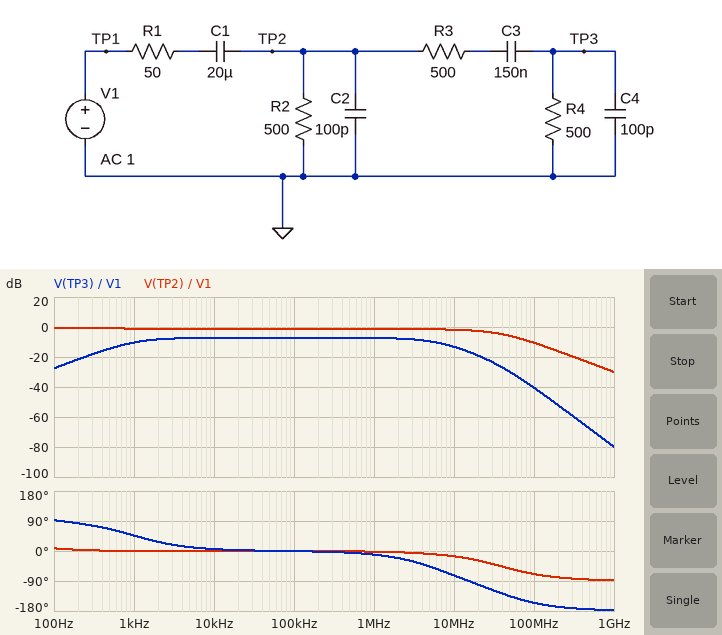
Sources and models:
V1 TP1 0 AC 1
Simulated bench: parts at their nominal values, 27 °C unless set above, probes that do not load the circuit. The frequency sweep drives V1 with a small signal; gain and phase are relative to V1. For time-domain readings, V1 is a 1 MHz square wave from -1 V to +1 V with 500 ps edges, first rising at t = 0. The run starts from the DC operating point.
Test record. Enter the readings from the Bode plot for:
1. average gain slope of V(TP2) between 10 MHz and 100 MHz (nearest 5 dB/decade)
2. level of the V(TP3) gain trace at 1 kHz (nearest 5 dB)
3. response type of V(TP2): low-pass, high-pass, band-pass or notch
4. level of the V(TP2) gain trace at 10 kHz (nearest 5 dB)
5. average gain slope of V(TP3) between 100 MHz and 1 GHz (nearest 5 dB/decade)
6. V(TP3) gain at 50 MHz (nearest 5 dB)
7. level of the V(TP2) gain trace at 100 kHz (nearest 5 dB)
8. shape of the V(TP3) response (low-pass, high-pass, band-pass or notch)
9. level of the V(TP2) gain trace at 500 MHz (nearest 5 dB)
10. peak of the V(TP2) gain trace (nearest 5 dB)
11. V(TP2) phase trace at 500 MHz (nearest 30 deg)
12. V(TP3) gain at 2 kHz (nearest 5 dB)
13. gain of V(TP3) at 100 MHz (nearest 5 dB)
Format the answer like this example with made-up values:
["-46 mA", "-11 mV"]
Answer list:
["-10 dB/decade", "-10 dB", "low-pass", "0 dB", "-40 dB/decade", "-30 dB", "0 dB", "band-pass", "-25 dB", "0 dB", "-90 deg", "-10 dB", "-40 dB"]
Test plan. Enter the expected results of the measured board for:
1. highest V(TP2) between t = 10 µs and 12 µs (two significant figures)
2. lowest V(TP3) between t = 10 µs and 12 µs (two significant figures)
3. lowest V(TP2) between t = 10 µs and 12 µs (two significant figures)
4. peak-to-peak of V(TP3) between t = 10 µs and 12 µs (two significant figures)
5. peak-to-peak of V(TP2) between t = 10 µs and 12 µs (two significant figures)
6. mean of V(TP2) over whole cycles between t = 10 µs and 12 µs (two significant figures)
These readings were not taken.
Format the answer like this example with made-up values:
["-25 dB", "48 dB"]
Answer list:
["1.7 V", "-33 mV", "1.3 mV", "870 mV", "1.7 V", "870 mV"]
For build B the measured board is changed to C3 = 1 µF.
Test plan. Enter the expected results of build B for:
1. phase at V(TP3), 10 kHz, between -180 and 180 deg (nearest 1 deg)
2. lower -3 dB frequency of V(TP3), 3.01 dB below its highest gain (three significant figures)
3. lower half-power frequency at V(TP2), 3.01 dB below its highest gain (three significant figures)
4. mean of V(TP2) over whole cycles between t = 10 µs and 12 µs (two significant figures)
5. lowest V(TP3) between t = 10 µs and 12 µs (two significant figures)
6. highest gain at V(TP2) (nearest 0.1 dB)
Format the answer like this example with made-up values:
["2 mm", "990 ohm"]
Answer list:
["1 deg", "160 Hz", "13.8 Hz", "870 mV", "-5.6 mV", "-1.2 dB"]
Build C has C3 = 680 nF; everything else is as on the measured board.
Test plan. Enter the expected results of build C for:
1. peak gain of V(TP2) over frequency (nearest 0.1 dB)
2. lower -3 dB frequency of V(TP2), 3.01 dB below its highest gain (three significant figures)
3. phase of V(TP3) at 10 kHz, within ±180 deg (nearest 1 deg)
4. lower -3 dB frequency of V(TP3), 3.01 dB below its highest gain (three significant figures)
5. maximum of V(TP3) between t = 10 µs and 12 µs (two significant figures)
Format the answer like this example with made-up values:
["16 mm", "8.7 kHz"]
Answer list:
["-1.2 dB", "13.8 Hz", "1 deg", "231 Hz", "860 mV"]
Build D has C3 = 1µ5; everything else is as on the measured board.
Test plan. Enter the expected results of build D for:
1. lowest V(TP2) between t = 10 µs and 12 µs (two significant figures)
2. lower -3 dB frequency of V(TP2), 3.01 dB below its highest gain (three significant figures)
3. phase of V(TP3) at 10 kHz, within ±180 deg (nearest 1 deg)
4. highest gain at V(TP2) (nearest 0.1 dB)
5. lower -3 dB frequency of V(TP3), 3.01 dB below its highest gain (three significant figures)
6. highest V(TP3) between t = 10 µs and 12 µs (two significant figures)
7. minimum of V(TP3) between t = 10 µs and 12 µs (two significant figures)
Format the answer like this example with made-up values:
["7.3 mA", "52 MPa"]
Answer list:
["-1.1 mV", "14.2 Hz", "1 deg", "-1.2 dB", "110 Hz", "870 mV", "-4.0 mV"]
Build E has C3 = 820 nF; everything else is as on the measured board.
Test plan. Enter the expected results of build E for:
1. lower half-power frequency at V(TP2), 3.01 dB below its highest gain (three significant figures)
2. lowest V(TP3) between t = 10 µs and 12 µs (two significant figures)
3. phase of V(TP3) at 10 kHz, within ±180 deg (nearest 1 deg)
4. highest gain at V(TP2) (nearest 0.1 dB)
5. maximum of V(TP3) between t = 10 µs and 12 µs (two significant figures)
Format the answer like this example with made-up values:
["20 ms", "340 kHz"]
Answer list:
["13.8 Hz", "-6.7 mV", "1 deg", "-1.2 dB", "860 mV"]
